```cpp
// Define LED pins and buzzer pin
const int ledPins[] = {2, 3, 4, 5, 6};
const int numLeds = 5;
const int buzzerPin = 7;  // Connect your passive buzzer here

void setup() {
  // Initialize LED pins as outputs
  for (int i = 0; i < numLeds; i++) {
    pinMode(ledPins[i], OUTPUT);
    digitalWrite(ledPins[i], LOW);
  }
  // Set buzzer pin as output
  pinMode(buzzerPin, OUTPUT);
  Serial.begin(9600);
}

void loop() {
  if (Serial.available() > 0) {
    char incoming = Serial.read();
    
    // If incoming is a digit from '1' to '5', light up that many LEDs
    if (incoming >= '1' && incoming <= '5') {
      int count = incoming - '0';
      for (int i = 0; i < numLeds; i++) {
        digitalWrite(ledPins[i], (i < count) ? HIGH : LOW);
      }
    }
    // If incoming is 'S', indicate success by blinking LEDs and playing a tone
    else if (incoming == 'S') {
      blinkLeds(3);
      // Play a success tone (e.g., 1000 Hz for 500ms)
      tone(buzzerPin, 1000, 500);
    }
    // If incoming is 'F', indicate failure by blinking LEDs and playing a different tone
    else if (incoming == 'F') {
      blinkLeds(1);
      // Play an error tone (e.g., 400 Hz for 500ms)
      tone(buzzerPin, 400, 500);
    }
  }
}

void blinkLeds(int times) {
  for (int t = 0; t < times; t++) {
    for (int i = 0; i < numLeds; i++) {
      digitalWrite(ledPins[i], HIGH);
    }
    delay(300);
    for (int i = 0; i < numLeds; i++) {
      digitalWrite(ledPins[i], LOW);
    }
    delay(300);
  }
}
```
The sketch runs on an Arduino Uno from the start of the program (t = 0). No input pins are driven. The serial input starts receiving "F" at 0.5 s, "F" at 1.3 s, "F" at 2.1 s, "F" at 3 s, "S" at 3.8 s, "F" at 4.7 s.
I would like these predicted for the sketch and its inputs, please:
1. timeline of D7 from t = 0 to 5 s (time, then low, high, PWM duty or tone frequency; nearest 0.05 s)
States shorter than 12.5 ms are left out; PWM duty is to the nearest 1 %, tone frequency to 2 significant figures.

0 s low; 1.1 s tone 400 Hz; 1.6 s low; 1.9 s tone 400 Hz; 2.4 s low; 2.7 s tone 400 Hz; 3.2 s low; 3.6 s tone 400 Hz; 4.1 s low
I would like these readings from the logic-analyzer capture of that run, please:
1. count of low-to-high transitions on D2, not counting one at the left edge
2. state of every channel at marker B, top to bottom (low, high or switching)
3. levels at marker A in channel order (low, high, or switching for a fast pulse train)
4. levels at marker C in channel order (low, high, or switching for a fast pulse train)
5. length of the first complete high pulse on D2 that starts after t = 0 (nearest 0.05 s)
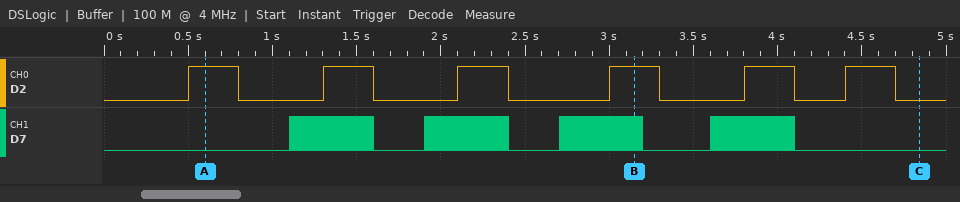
6
D2 high, D7 switching
D2 high, D7 low
D2 low, D7 low
0.30 s
